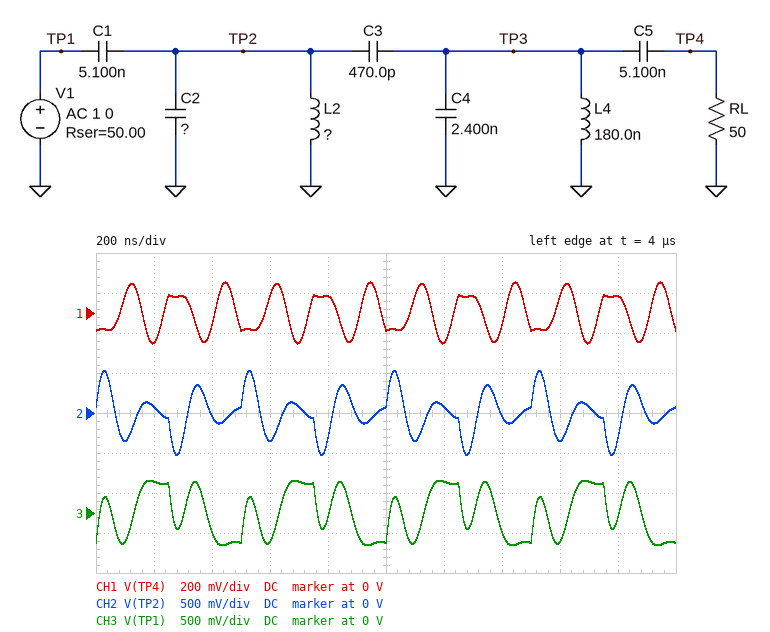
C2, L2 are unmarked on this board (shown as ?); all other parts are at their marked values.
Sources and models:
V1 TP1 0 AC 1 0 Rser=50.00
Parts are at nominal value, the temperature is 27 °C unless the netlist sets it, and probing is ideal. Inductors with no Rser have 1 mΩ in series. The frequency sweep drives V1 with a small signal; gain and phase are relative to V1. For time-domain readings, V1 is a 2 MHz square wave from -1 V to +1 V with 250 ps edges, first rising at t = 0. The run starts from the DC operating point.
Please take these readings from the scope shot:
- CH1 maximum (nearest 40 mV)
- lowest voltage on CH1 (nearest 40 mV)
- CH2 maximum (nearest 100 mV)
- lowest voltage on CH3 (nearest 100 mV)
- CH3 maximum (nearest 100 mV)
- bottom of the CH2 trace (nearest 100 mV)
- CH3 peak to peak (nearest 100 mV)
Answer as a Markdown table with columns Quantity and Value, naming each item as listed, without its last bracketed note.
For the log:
| Quantity | Value |
|---|---|
| CH1 maximum | 160 mV |
| lowest voltage on CH1 | -160 mV |
| CH2 maximum | 500 mV |
| lowest voltage on CH3 | -400 mV |
| CH3 maximum | 400 mV |
| bottom of the CH2 trace | -500 mV |
| CH3 peak to peak | 800 mV |
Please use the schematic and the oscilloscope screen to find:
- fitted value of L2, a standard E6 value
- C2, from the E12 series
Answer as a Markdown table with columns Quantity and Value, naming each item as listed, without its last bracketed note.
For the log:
| Quantity | Value |
|---|---|
| fitted value of L2, a standard E6 value | 330 nH |
| C2, from the E12 series | 1 nF |
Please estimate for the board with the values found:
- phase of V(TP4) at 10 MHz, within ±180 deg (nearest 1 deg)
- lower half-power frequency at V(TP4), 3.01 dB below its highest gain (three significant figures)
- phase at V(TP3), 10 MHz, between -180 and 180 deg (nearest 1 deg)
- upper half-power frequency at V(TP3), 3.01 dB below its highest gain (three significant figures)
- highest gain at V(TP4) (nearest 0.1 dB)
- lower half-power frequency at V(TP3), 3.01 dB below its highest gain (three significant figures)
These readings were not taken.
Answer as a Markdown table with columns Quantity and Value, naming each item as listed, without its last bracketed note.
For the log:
| Quantity | Value |
|---|---|
| phase of V(TP4) at 10 MHz, within ±180 deg | -40 deg |
| lower half-power frequency at V(TP4), 3.01 dB below its highest gain | 6.14 MHz |
| phase at V(TP3), 10 MHz, between -180 and 180 deg | -43 deg |
| upper half-power frequency at V(TP3), 3.01 dB below its highest gain | 8.42 MHz |
| highest gain at V(TP4) | -6.0 dB |
| lower half-power frequency at V(TP3), 3.01 dB below its highest gain | 6.14 MHz |
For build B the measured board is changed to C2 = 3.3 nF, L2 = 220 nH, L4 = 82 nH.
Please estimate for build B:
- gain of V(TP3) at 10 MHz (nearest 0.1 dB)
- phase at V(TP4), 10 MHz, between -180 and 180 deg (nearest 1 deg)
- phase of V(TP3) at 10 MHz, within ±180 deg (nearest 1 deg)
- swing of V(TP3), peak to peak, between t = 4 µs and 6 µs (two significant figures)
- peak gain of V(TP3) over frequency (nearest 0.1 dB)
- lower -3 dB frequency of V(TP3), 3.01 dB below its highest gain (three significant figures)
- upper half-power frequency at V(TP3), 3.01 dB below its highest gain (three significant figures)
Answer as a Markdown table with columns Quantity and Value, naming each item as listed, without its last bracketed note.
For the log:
| Quantity | Value |
|---|---|
| gain of V(TP3) at 10 MHz | -17.7 dB |
| phase at V(TP4), 10 MHz, between -180 and 180 deg | 55 deg |
| phase of V(TP3) at 10 MHz, within ±180 deg | 51 deg |
| swing of V(TP3), peak to peak, between t = 4 µs and 6 µs | 120 mV |
| peak gain of V(TP3) over frequency | -15.6 dB |
| lower -3 dB frequency of V(TP3), 3.01 dB below its highest gain | 9.87 MHz |
| upper half-power frequency at V(TP3), 3.01 dB below its highest gain | 11.0 MHz |
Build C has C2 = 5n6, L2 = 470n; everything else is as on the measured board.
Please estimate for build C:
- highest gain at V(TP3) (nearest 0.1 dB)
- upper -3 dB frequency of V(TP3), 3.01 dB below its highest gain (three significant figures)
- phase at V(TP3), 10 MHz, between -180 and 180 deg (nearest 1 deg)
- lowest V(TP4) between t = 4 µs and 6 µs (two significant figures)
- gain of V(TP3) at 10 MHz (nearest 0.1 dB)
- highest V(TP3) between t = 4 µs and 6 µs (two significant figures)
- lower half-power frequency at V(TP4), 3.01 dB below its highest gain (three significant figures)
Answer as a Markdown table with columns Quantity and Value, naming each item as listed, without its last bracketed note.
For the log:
| Quantity | Value |
|---|---|
| highest gain at V(TP3) | -20.6 dB |
| upper -3 dB frequency of V(TP3), 3.01 dB below its highest gain | 7.56 MHz |
| phase at V(TP3), 10 MHz, between -180 and 180 deg | -71 deg |
| lowest V(TP4) between t = 4 µs and 6 µs | -24 mV |
| gain of V(TP3) at 10 MHz | -34.8 dB |
| highest V(TP3) between t = 4 µs and 6 µs | 25 mV |
| lower half-power frequency at V(TP4), 3.01 dB below its highest gain | 6.43 MHz |
